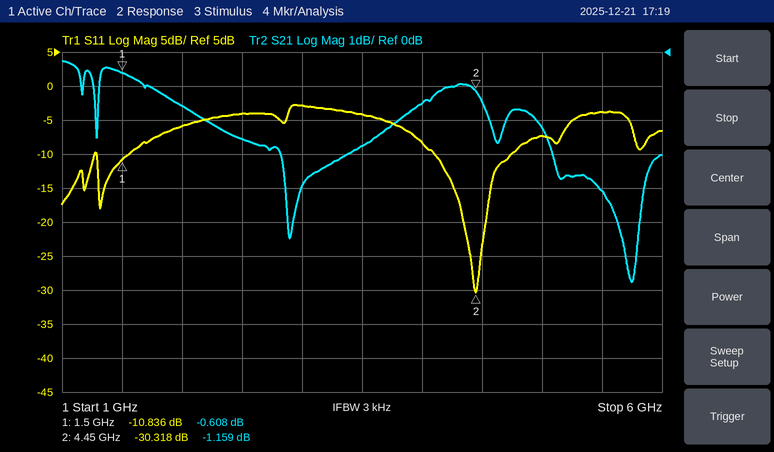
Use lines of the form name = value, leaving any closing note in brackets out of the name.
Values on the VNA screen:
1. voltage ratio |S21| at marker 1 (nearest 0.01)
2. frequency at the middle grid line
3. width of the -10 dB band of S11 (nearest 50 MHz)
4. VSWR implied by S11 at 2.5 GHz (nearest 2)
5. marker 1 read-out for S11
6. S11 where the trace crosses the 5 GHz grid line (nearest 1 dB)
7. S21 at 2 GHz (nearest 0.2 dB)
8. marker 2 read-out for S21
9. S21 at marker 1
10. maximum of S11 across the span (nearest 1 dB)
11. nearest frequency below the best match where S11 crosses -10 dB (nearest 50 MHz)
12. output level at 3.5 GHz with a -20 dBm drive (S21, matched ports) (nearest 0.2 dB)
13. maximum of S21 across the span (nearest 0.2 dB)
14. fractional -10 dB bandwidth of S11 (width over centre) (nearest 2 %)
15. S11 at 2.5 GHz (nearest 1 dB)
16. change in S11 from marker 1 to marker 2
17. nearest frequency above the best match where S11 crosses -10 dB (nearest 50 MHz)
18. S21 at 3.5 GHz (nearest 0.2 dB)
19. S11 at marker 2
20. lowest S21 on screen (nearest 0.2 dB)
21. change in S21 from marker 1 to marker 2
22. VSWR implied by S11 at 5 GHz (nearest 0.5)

voltage ratio |S21| at marker 1 = 0.93
frequency at the middle grid line = 3.5 GHz
width of the -10 dB band of S11 = 650 MHz
VSWR implied by S11 at 2.5 GHz = 4
marker 1 read-out for S11 = -10.836 dB
S11 where the trace crosses the 5 GHz grid line = -7 dB
S21 at 2 GHz = -1.6 dB
marker 2 read-out for S21 = -1.159 dB
S21 at marker 1 = -0.608 dB
maximum of S11 across the span = -3 dB
nearest frequency below the best match where S11 crosses -10 dB = 4.10 GHz
output level at 3.5 GHz with a -20 dBm drive (S21, matched ports) = -22.8 dBm
maximum of S21 across the span = -0.2 dB
fractional -10 dB bandwidth of S11 (width over centre) = 14 %
S11 at 2.5 GHz = -4 dB
change in S11 from marker 1 to marker 2 = -19.482 dB
nearest frequency above the best match where S11 crosses -10 dB = 4.75 GHz
S21 at 3.5 GHz = -2.8 dB
S11 at marker 2 = -30.318 dB
lowest S21 on screen = -6.8 dB
change in S21 from marker 1 to marker 2 = -0.551 dB
VSWR implied by S11 at 5 GHz = 2.5
